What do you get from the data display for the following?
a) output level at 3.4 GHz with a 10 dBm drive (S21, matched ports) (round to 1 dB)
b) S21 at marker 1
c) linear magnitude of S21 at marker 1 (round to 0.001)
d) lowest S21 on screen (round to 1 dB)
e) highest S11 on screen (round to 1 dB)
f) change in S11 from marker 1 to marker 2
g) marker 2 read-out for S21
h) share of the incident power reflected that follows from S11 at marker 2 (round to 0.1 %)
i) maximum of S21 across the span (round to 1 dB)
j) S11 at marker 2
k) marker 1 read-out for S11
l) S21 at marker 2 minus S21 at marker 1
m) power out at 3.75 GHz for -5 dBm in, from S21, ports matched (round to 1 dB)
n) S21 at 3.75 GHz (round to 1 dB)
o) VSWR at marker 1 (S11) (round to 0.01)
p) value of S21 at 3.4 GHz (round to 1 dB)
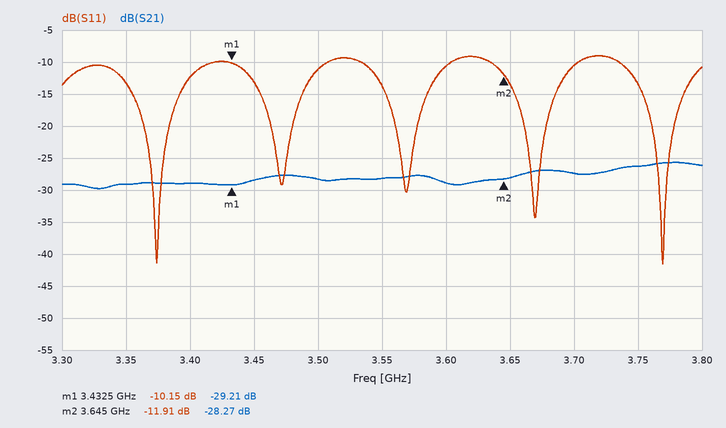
-19 dBm
-29.21 dB
0.035
-30 dB
-9 dB
-1.76 dB
-28.27 dB
6.4 %
-26 dB
-11.91 dB
-10.15 dB
0.94 dB
-31 dBm
-26 dB
1.90
-29 dB
